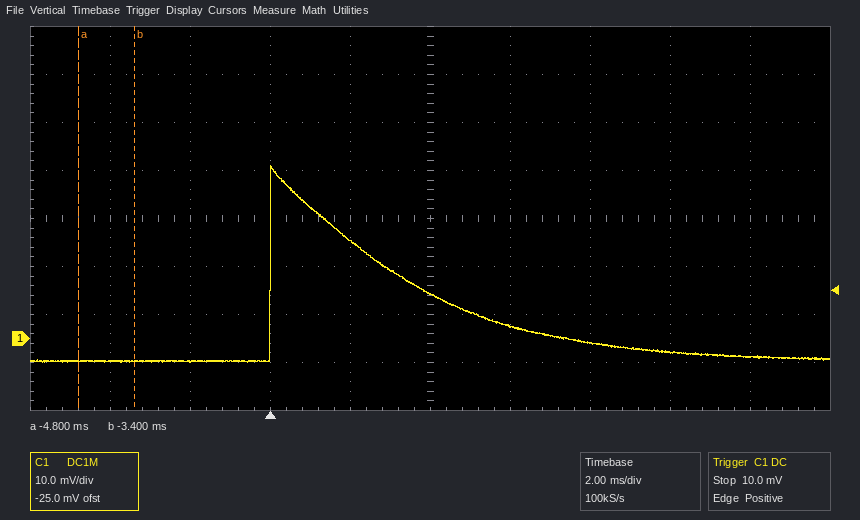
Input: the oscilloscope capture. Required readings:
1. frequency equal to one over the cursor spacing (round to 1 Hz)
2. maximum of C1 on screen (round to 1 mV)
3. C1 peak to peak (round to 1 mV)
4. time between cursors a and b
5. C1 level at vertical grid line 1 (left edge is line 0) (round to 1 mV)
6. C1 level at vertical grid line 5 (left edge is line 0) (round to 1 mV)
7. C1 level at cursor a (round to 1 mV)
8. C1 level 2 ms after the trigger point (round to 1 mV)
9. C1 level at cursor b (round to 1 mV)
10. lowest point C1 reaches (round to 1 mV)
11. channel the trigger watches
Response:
714 Hz
36 mV
41 mV
1.4 ms
-5 mV
9 mV
-5 mV
20 mV
-5 mV
-5 mV
C1
